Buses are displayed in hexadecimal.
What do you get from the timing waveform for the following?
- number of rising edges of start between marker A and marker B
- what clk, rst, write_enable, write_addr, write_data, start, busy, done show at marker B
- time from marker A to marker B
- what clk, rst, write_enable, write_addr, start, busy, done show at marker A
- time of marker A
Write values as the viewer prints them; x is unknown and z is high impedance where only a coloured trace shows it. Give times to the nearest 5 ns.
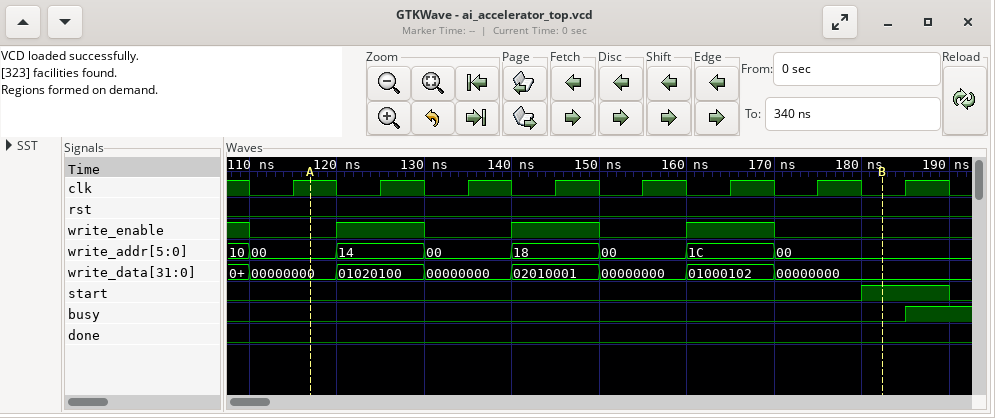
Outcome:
1
clk=0, rst=0, write_enable=0, write_addr=00, write_data=00000000, start=1, busy=0, done=0
65 ns
clk=1, rst=0, write_enable=0, write_addr=00, start=0, busy=0, done=0
115 ns
